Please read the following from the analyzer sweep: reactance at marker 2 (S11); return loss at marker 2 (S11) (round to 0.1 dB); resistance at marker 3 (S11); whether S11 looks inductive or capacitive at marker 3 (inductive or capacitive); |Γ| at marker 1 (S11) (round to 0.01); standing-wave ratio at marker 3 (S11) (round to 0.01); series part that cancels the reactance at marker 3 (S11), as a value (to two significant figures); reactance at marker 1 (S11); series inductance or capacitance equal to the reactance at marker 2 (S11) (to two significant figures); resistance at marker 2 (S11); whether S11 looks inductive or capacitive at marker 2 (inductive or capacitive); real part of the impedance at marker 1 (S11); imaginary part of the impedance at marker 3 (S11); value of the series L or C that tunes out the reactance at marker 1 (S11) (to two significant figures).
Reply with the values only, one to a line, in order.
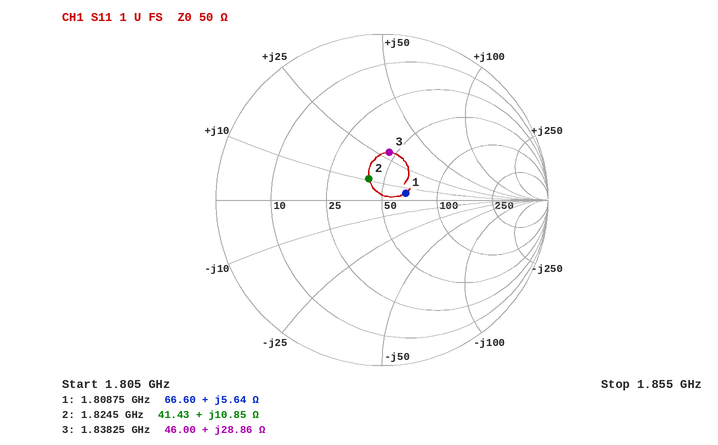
+10.85 Ω
16.5 dB
46.00 Ω
inductive
0.15
1.82
3.0 pF
+5.64 Ω
950 pH
41.43 Ω
inductive
66.60 Ω
+28.86 Ω
16 pF
